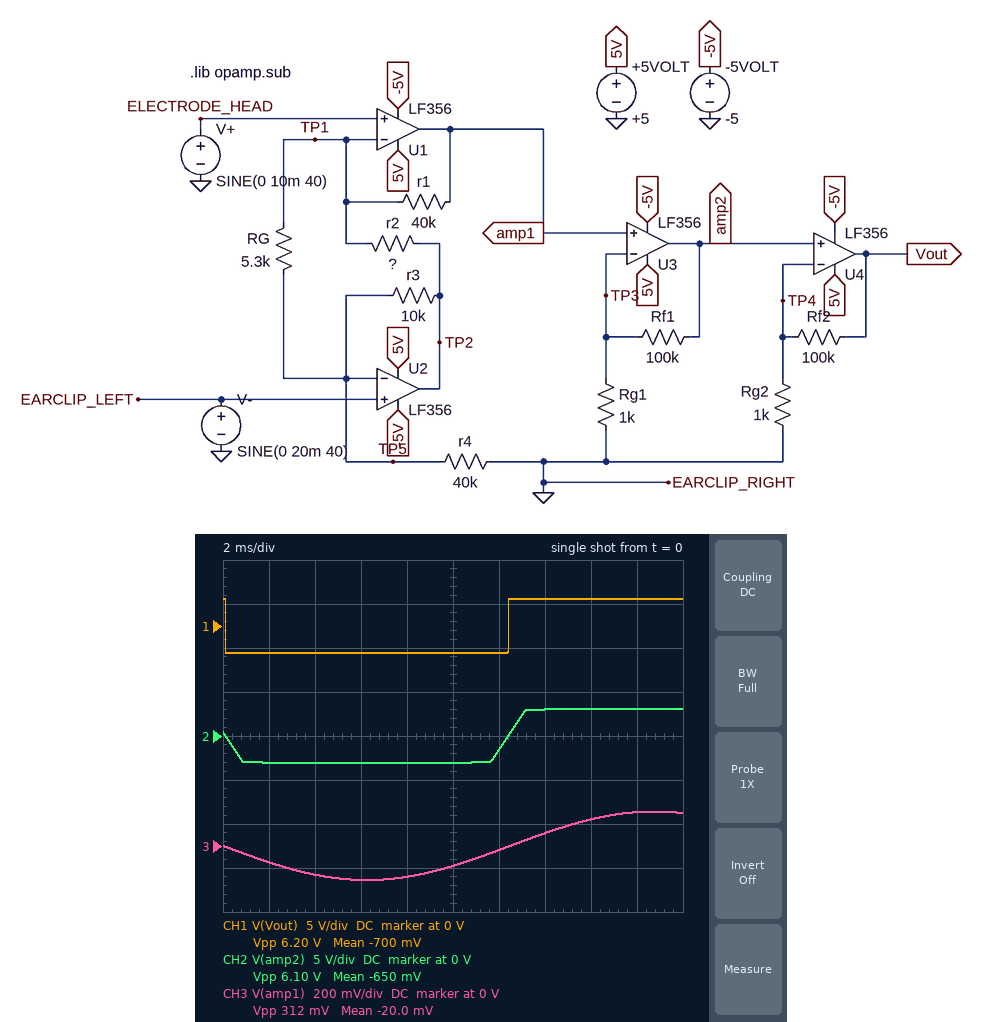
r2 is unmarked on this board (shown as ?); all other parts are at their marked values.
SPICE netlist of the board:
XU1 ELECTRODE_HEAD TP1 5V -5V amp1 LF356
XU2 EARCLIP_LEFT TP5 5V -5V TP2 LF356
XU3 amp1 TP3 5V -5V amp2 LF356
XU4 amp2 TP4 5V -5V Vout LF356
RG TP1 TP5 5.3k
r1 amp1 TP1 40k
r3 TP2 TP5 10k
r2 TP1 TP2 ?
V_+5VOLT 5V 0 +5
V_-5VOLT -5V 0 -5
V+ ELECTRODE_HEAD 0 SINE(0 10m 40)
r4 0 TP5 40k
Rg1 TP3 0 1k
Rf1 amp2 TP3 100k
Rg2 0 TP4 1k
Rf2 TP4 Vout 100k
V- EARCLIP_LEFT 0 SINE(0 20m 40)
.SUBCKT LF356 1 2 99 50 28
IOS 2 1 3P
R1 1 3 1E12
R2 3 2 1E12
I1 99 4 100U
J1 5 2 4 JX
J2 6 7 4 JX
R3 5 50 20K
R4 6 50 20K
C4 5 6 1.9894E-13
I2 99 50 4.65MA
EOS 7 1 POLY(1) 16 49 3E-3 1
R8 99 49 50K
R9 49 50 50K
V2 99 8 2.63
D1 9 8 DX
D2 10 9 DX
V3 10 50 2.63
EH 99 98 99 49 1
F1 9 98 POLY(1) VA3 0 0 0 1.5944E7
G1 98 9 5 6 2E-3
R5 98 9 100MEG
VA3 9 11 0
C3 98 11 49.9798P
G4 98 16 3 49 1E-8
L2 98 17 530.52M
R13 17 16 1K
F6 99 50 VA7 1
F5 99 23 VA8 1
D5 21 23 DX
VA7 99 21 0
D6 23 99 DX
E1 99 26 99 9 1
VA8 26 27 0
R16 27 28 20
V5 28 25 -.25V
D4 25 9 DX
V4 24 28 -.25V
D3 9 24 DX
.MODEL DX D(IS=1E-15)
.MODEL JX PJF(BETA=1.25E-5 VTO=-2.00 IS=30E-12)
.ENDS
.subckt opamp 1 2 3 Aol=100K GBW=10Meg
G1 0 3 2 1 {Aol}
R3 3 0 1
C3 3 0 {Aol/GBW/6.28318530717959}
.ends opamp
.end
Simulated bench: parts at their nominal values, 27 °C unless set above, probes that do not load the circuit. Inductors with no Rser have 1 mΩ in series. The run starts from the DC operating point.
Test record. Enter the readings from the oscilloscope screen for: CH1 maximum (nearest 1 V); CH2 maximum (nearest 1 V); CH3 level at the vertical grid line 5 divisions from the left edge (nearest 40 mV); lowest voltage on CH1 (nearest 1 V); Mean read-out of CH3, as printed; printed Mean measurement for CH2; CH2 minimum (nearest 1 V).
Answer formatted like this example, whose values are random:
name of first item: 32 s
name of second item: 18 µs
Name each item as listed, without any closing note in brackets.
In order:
CH1 maximum: 3 V
CH2 maximum: 3 V
CH3 level at the vertical grid line 5 divisions from the left edge: -80 mV
lowest voltage on CH1: -3 V
Mean read-out of CH3, as printed: -20.0 mV
printed Mean measurement for CH2: -650 mV
CH2 minimum: -3 V
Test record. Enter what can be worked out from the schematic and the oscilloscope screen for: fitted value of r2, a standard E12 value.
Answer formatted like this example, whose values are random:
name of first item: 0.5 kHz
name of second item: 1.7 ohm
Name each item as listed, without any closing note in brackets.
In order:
fitted value of r2, a standard E12 value: 15 kΩ
